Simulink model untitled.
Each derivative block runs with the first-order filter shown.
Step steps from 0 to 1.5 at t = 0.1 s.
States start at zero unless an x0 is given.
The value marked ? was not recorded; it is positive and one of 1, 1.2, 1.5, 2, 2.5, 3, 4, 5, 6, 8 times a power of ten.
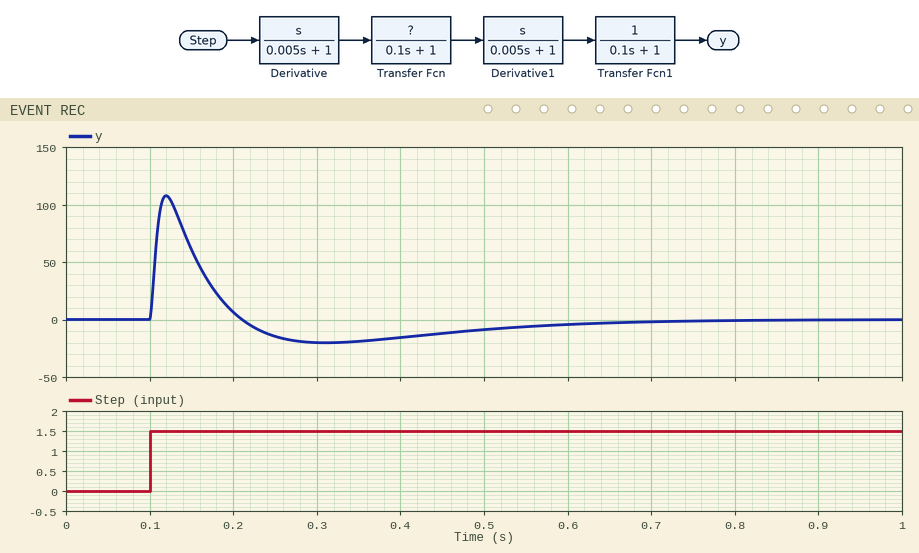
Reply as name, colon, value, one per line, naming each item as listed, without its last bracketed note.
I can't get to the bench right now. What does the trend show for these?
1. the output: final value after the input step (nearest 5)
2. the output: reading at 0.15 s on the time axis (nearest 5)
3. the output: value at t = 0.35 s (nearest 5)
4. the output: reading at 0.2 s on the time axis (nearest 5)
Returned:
the output: final value after the input step: 0
the output: reading at 0.15 s on the time axis: 60
the output: value at t = 0.35 s: -20
the output: reading at 0.2 s on the time axis: 5
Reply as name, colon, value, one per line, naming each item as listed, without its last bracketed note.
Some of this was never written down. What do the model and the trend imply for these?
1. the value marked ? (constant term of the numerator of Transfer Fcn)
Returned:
the value marked ?: 1
